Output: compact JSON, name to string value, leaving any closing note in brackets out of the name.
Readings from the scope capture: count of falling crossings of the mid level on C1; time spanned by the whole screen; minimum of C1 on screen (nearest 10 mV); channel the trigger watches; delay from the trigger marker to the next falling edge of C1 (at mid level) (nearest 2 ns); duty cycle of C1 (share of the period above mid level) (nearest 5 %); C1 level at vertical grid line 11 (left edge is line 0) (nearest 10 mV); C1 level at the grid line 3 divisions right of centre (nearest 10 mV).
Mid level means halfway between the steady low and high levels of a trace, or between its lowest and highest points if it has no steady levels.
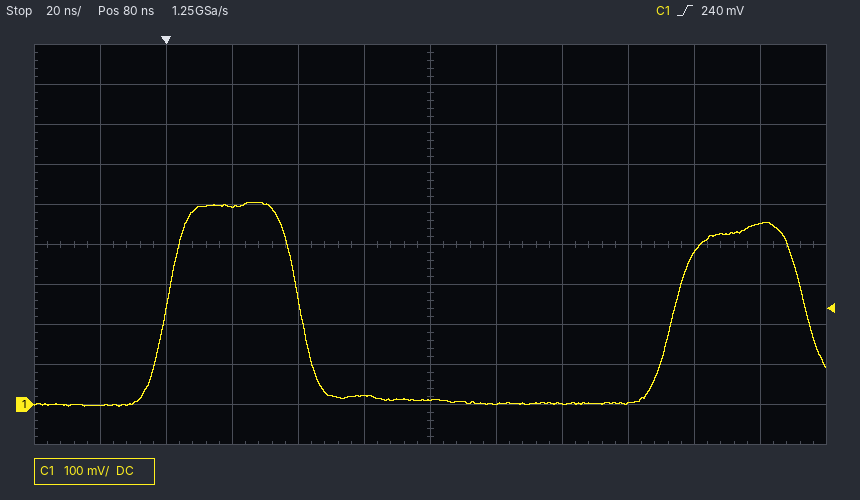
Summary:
{"count of falling crossings of the mid level on C1": "2", "time spanned by the whole screen": "240 ns", "minimum of C1 on screen": "0 mV", "channel the trigger watches": "C1", "delay from the trigger marker to the next falling edge of C1 (at mid level)": "40 ns", "duty cycle of C1 (share of the period above mid level)": "25 %", "C1 level at vertical grid line 11 (left edge is line 0)": "450 mV", "C1 level at the grid line 3 divisions right of centre": "0 mV"}
